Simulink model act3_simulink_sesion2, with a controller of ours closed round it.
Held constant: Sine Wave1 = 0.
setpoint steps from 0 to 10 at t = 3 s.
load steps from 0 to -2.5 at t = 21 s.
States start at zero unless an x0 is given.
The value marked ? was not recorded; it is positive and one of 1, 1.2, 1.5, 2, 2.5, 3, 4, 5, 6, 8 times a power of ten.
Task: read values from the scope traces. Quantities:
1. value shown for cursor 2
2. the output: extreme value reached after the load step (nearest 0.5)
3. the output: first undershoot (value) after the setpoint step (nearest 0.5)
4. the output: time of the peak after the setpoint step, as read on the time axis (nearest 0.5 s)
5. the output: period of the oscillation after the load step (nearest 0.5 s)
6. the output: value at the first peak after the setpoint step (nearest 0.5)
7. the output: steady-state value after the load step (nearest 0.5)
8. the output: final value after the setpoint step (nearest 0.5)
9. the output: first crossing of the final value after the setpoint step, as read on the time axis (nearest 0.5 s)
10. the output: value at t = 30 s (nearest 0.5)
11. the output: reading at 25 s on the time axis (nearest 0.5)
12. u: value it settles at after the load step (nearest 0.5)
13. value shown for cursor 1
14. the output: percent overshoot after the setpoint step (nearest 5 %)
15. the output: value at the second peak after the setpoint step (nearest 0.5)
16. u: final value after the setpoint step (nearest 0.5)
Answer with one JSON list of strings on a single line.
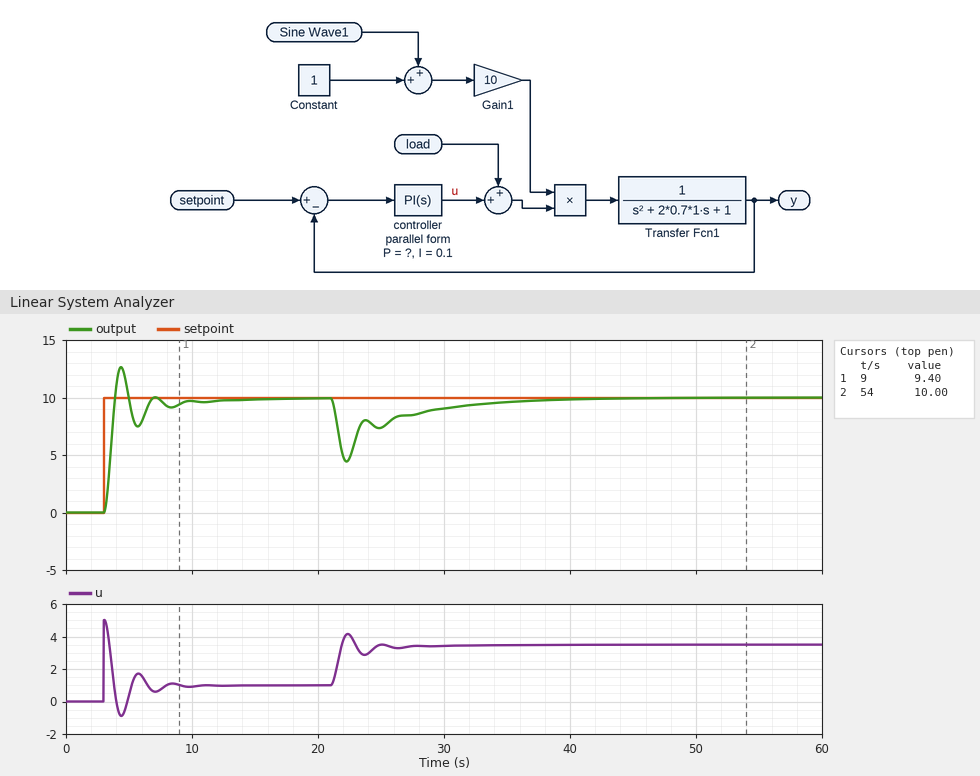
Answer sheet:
["10.00", "4.5", "7.5", "4.5 s", "2.5 s", "12.5", "10.0", "10.0", "4.0 s", "9.0", "7.5", "3.5", "9.40", "25 %", "10.0", "1.0"]
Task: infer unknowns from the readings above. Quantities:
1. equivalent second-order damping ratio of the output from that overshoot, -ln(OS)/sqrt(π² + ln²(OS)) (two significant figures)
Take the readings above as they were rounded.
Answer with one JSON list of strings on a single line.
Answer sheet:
["0.40"]
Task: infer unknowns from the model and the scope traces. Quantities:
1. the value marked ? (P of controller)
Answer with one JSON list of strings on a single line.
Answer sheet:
["0.5"]
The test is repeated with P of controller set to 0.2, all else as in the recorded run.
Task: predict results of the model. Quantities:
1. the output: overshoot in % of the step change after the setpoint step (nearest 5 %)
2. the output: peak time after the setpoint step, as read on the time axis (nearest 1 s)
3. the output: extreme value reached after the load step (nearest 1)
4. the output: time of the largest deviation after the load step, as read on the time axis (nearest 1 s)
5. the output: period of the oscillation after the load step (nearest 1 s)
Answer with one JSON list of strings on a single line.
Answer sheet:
["15 %", "5 s", "1", "23 s", "4 s"]
